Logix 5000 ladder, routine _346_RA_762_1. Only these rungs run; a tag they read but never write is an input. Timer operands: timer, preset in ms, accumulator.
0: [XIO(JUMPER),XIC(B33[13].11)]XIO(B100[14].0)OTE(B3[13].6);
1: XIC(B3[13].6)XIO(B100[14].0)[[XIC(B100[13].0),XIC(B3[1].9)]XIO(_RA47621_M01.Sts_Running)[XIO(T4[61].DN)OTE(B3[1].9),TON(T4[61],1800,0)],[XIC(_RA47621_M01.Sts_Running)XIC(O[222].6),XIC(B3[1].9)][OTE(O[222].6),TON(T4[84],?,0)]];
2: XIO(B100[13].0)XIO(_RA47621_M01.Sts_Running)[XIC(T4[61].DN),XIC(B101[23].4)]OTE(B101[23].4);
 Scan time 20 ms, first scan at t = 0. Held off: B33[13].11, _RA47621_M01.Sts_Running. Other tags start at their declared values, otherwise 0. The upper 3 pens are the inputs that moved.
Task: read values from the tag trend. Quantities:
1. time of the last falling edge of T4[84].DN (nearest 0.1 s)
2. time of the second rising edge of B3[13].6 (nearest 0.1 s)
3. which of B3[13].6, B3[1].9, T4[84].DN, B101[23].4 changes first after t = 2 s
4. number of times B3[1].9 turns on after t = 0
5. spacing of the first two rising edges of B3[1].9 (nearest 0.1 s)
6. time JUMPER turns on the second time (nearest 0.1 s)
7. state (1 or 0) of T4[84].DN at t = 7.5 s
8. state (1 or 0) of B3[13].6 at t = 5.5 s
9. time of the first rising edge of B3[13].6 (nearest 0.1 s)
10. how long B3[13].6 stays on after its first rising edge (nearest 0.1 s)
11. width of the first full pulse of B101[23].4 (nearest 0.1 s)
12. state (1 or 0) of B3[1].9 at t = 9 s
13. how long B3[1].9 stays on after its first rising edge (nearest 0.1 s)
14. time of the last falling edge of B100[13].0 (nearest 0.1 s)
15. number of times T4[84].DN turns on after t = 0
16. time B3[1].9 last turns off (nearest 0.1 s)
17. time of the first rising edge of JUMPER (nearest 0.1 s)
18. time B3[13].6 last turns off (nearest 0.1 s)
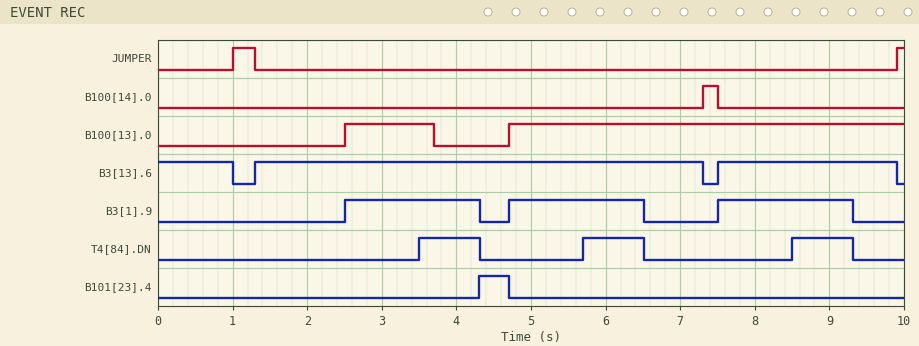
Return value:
9.3 s
7.5 s
B3[1].9
3
2.2 s
9.9 s
0
1
1.3 s
6.0 s
0.4 s
1
1.8 s
3.7 s
3
9.3 s
1.0 s
9.9 s
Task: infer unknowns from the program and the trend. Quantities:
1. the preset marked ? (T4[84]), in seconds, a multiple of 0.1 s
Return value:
1.0 s
